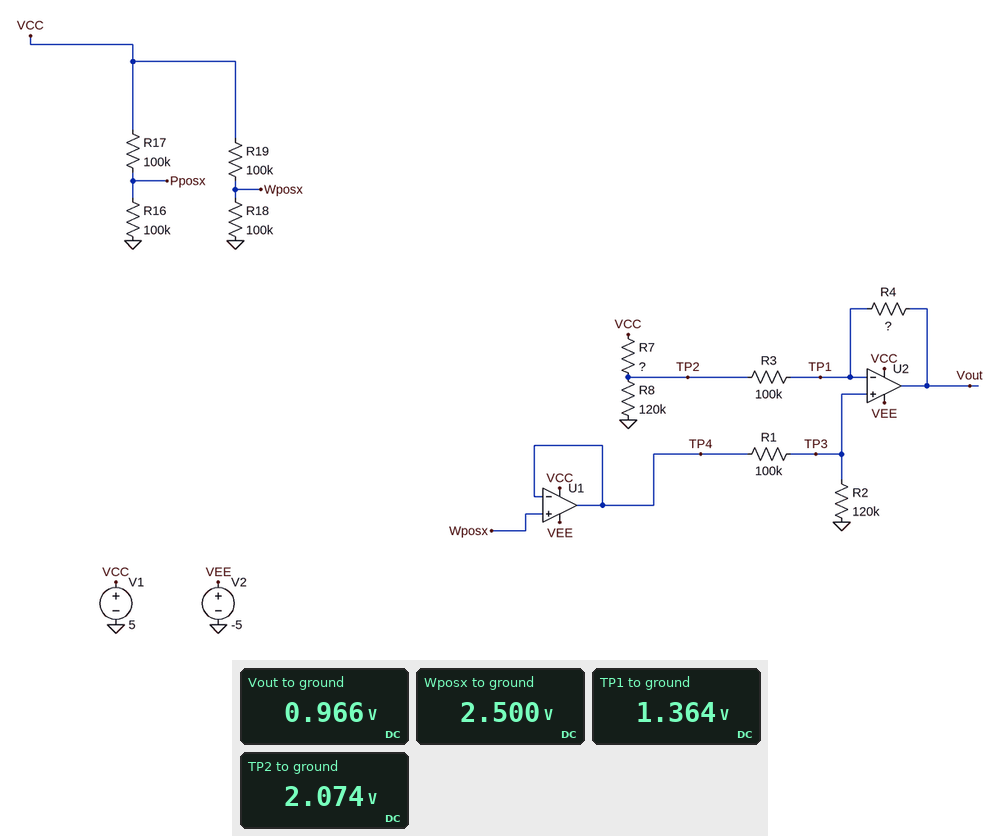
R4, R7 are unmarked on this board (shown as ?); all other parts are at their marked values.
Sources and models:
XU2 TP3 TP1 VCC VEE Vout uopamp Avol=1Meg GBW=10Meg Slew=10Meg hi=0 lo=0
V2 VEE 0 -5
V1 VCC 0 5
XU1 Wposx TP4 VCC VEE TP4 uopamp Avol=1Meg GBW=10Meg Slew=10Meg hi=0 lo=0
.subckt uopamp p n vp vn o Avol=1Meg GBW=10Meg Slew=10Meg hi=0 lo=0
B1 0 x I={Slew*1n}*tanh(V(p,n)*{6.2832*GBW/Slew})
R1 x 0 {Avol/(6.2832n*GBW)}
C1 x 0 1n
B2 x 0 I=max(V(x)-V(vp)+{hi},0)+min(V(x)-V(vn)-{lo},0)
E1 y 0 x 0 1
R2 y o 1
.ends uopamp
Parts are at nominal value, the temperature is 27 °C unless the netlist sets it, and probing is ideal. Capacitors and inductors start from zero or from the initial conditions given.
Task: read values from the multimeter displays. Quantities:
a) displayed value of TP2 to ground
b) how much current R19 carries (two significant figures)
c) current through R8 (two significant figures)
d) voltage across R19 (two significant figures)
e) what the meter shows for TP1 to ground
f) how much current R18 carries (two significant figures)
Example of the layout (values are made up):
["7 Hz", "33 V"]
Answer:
["2.074 V", "25 µA", "17 µA", "2.5 V", "1.364 V", "25 µA"]
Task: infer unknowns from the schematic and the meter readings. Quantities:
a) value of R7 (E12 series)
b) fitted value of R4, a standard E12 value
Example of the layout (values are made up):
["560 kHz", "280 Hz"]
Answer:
["120 kΩ", "56 kΩ"]
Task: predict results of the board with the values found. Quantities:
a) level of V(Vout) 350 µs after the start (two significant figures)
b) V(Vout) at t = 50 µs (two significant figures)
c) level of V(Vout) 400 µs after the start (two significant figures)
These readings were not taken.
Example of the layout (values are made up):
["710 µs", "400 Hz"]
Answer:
["970 mV", "970 mV", "970 mV"]
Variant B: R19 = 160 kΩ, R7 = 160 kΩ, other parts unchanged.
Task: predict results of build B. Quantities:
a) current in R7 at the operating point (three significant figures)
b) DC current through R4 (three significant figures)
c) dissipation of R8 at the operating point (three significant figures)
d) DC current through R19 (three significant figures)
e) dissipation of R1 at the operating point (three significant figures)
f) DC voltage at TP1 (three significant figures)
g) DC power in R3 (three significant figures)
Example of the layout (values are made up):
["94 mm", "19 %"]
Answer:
["20.6 µA", "6.49 µA", "24.0 µW", "19.2 µA", "7.64 µW", "1.05 V", "4.21 µW"]
